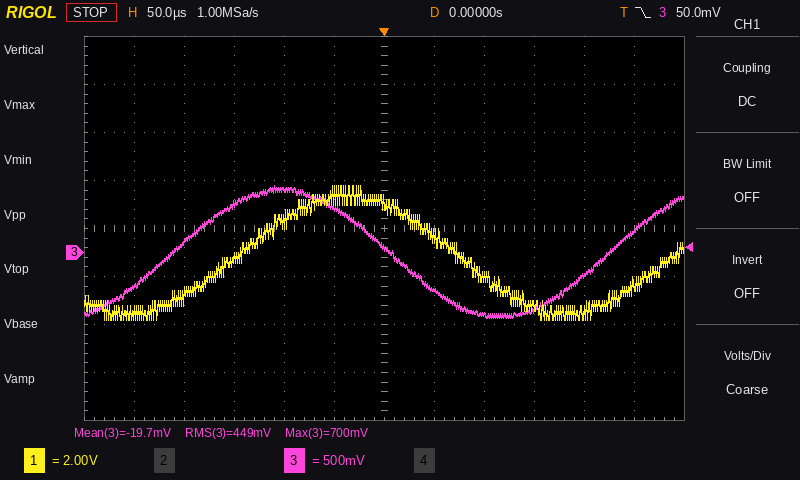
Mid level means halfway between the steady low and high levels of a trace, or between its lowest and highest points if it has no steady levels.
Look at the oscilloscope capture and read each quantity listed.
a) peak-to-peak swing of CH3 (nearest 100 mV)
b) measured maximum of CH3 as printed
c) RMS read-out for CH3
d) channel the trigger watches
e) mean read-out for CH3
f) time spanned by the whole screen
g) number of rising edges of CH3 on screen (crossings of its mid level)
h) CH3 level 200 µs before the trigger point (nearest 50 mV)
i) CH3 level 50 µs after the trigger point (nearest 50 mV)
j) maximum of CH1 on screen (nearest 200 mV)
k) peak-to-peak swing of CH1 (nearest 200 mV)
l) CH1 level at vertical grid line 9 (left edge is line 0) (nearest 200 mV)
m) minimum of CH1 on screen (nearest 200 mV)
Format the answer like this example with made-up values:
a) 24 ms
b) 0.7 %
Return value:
a) 1.40 V
b) 700 mV
c) 449 mV
d) CH3
e) -19.7 mV
f) 600 µs
g) 2
h) 100 mV
i) -400 mV
j) 2.8 V
k) 5.6 V
l) -2.2 V
m) -2.8 V
